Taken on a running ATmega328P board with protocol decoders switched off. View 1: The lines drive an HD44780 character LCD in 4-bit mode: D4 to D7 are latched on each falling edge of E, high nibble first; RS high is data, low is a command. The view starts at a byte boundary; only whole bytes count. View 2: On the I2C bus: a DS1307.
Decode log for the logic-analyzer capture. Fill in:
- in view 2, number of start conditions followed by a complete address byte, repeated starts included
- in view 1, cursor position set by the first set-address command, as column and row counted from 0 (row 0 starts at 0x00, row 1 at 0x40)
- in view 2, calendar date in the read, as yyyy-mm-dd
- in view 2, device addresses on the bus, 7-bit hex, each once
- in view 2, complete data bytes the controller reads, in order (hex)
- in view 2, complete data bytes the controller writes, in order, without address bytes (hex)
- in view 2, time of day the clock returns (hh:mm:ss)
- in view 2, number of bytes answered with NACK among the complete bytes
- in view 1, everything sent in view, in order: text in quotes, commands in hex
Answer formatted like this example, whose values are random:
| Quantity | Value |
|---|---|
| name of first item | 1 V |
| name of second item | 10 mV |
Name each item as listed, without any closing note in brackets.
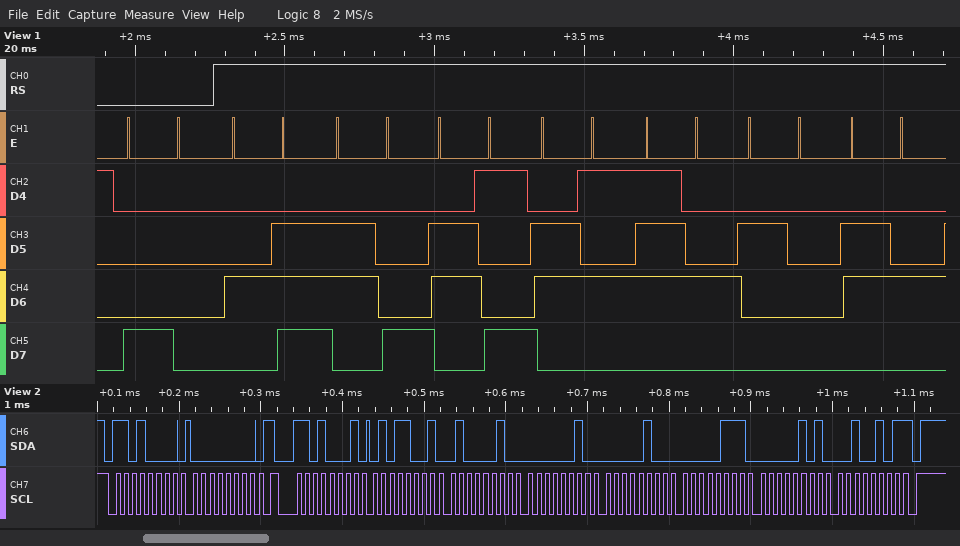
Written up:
| Quantity | Value |
|---|---|
| in view 2, number of start conditions followed by a complete address byte, repeated starts included | 2 |
| in view 1, cursor position set by the first set-address command, as column and row counted from 0 | column 0, row 0 |
| in view 2, calendar date in the read, as yyyy-mm-dd | 2025-05-07 |
| in view 2, device addresses on the bus, 7-bit hex, each once | 0x68 |
| in view 2, complete data bytes the controller reads, in order | 59 42 02 04 07 05 25 |
| in view 2, complete data bytes the controller writes, in order, without address bytes | 00 |
| in view 2, time of day the clock returns | 02:42:59 |
| in view 2, number of bytes answered with NACK among the complete bytes | 1 |
| in view 1, everything sent in view, in order: text in quotes, commands in hex | 0x80 "Nhiet d" |
